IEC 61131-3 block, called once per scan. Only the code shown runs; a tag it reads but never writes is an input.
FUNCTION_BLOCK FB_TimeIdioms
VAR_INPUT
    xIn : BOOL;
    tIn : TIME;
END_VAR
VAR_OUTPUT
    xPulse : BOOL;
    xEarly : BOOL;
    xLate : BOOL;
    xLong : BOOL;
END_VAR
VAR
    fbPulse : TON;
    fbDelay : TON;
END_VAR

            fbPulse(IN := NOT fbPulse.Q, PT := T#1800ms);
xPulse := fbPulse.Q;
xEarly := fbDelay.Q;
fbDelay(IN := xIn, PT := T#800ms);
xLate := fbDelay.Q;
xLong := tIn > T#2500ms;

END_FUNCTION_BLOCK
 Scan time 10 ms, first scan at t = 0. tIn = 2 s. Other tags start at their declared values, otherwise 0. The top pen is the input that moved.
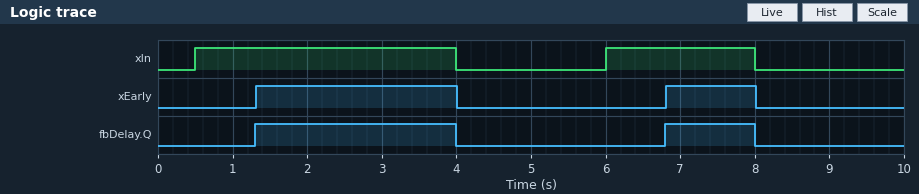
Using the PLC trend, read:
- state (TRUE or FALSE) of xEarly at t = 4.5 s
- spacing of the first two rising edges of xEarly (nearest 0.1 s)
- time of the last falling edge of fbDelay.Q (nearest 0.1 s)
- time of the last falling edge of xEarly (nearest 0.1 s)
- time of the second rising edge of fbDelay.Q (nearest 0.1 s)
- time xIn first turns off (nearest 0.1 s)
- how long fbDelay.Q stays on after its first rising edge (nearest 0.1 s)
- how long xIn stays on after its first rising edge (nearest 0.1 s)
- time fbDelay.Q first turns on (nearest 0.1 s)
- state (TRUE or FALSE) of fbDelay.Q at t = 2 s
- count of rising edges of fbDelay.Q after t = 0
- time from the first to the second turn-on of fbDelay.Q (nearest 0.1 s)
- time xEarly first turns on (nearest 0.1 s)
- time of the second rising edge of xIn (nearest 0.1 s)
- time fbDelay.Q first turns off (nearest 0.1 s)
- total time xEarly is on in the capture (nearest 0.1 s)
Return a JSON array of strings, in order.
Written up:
["FALSE", "5.5 s", "8.0 s", "8.0 s", "6.8 s", "4.0 s", "2.7 s", "3.5 s", "1.3 s", "TRUE", "2", "5.5 s", "1.3 s", "6.0 s", "4.0 s", "3.9 s"]
